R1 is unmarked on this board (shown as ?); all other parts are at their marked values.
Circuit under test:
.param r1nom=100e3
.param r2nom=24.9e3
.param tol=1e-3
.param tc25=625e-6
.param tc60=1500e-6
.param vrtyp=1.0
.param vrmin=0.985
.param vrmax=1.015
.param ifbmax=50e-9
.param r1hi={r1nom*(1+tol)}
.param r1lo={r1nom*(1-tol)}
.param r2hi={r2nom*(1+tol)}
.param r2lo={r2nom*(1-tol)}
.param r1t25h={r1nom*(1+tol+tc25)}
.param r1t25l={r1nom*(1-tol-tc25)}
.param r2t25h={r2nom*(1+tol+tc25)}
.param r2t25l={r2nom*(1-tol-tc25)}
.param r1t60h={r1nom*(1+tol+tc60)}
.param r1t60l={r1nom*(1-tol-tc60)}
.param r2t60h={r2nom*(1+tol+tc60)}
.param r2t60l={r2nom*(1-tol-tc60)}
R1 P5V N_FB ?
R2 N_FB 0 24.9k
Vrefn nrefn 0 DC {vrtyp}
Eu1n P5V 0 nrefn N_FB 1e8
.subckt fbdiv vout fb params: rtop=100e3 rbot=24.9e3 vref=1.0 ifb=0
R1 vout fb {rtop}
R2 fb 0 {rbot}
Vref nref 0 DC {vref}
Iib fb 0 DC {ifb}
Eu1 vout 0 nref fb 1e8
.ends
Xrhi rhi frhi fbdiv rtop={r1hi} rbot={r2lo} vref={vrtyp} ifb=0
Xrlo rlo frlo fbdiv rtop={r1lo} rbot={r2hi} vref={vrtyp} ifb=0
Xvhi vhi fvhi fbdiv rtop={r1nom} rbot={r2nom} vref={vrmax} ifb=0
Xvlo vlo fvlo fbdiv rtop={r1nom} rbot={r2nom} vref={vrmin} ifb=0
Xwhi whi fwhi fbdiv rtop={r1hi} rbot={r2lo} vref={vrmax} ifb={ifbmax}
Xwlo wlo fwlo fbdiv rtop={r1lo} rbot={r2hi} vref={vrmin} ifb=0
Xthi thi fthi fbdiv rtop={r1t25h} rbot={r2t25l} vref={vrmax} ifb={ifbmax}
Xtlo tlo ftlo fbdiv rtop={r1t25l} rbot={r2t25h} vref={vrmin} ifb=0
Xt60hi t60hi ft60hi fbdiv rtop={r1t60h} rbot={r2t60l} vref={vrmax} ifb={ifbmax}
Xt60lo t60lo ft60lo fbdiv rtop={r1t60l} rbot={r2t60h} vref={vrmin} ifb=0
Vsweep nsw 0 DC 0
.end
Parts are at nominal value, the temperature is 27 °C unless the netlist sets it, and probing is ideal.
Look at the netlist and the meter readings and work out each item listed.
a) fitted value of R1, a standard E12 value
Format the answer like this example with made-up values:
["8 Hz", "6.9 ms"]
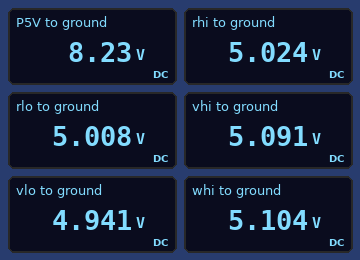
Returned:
["180 kΩ"]
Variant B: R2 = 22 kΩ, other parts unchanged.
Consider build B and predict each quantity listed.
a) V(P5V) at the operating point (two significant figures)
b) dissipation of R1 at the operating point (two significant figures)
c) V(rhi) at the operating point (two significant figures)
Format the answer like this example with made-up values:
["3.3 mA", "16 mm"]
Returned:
["9.2 V", "370 µW", "5.0 V"]
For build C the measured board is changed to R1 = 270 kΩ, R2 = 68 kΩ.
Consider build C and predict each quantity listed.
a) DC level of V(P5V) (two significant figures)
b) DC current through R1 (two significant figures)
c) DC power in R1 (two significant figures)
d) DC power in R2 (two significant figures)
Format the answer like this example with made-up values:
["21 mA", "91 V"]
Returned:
["5.0 V", "15 µA", "58 µW", "15 µW"]
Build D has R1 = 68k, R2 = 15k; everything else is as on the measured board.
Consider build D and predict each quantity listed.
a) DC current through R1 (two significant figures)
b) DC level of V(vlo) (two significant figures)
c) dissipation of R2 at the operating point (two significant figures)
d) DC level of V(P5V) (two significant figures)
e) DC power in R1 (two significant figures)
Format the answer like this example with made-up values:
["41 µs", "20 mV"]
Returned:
["67 µA", "4.9 V", "67 µW", "5.5 V", "300 µW"]
